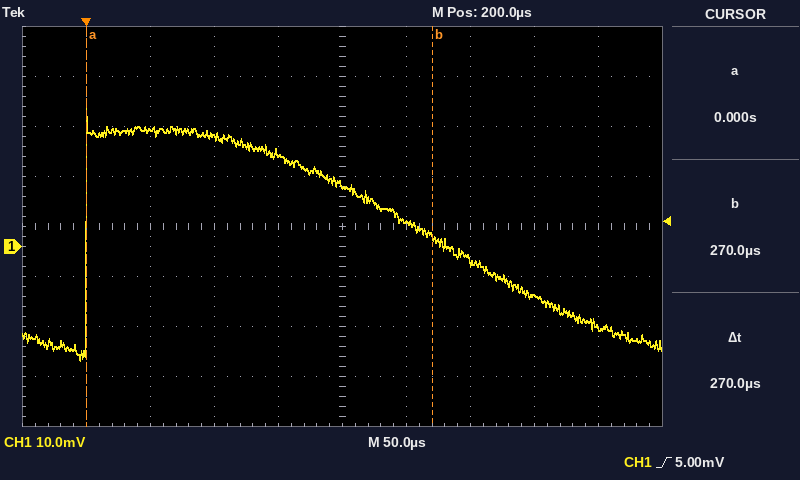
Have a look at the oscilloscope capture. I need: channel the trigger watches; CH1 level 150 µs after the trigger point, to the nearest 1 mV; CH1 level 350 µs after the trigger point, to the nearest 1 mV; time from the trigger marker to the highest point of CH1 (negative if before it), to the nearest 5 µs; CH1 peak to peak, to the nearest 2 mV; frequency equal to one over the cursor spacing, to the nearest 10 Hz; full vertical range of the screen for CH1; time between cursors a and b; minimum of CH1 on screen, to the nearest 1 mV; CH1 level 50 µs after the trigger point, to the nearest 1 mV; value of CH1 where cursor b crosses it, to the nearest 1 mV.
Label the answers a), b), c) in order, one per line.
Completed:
a) CH1
b) 19 mV
c) -10 mV
d) 0 µs
e) 50 mV
f) 3.70 kHz
g) 80 mV
h) 270 µs
i) -23 mV
j) 23 mV
k) 2 mV
